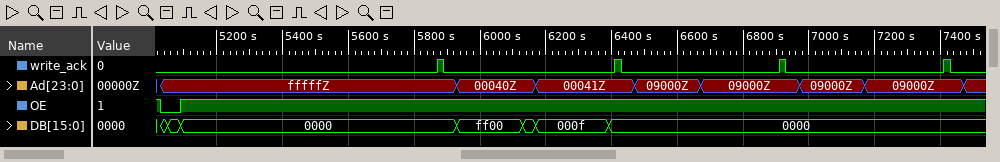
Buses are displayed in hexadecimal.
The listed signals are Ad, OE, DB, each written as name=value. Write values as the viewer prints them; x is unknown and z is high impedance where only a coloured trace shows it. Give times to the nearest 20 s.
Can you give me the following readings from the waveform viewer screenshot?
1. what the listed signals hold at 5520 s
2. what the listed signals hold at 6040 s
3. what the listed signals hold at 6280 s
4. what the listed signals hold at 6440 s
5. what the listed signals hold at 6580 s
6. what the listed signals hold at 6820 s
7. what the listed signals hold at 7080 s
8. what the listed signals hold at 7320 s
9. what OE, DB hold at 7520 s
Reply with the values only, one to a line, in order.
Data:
Ad=fffffZ, OE=1, DB=0000
Ad=00040Z, OE=1, DB=ff00
Ad=00041Z, OE=1, DB=000f
Ad=00041Z, OE=1, DB=0000
Ad=09000Z, OE=1, DB=0000
Ad=09000Z, OE=1, DB=0000
Ad=09000Z, OE=1, DB=0000
Ad=09000Z, OE=1, DB=0000
OE=1, DB=0000
